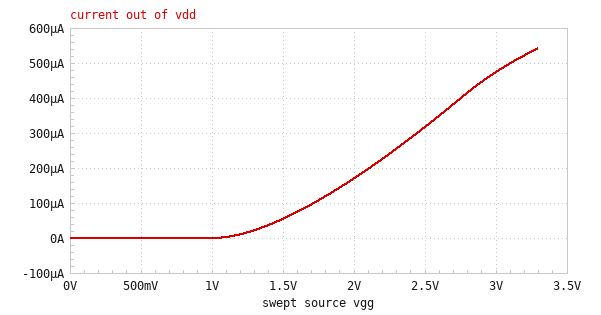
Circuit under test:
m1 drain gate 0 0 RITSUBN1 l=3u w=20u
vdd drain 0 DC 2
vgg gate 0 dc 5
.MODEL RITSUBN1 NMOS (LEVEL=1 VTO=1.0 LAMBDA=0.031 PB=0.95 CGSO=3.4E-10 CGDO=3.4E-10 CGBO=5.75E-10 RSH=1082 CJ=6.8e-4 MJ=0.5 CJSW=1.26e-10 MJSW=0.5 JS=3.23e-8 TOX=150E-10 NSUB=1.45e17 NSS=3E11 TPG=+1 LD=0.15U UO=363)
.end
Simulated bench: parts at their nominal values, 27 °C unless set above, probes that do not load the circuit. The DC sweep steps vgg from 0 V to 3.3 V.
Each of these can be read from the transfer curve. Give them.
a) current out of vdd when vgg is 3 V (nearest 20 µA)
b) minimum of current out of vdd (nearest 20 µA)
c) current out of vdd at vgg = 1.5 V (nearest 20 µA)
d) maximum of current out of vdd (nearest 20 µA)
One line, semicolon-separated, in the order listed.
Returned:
480 µA; 0 A; 60 µA; 540 µA
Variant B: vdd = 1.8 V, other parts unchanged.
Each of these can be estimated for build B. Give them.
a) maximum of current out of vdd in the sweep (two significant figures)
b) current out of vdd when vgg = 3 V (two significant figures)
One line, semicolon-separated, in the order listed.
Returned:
510 µA; 450 µA
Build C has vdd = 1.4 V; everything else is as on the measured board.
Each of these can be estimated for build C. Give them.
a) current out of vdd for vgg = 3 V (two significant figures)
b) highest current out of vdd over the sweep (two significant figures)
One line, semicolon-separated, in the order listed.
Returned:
390 µA; 420 µA
